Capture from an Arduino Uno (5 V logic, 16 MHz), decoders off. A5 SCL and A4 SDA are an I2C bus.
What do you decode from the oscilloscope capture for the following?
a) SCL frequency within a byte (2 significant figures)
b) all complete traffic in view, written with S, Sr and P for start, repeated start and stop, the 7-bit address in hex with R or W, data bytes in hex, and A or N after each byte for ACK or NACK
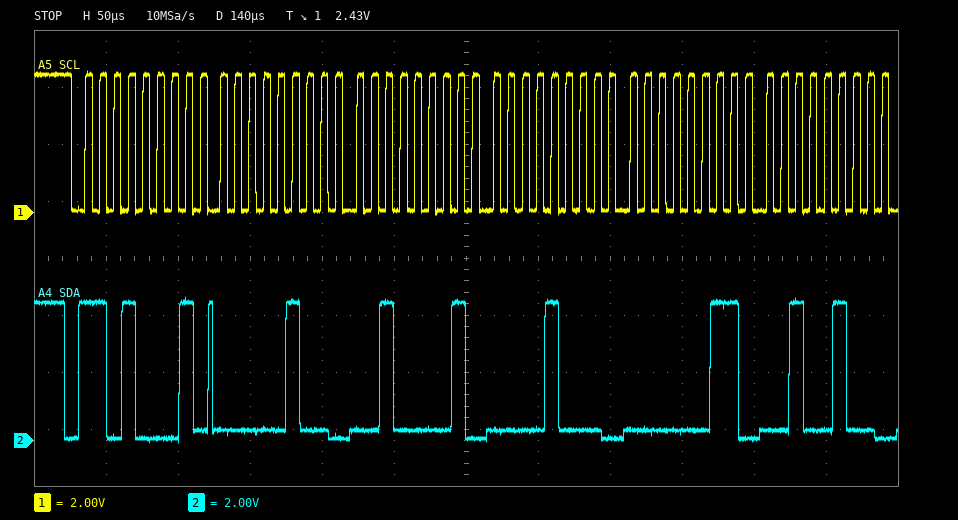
100 kHz
S 68R A 04 A 21 A 08 A 03 A 24 A
